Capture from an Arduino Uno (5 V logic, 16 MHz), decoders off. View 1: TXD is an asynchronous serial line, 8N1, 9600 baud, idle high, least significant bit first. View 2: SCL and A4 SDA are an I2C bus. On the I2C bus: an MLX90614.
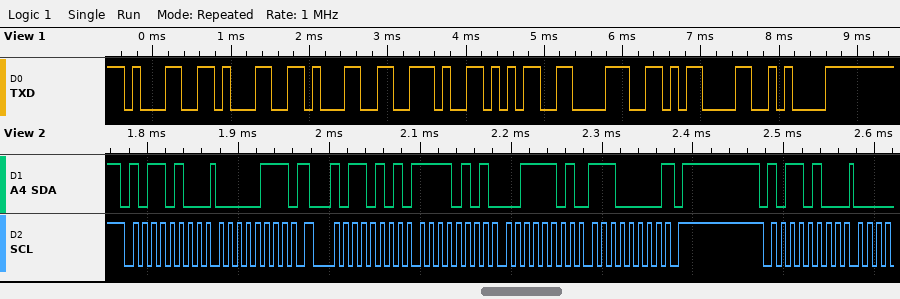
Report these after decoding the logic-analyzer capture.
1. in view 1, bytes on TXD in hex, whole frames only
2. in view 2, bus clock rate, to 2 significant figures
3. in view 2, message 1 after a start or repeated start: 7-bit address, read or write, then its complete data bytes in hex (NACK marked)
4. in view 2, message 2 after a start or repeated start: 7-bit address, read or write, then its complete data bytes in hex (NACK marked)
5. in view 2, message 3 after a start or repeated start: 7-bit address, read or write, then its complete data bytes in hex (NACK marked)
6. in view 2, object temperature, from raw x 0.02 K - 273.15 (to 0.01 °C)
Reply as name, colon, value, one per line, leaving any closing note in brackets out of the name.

in view 1, bytes on TXD in hex, whole frames only: 31 31 31 2E 35 38 0D 0A
in view 2, bus clock rate, to 2 significant figures: 100 kHz
in view 2, message 1 after a start or repeated start: 7-bit address, read or write, then its complete data bytes in hex: 0x5A write: 07
in view 2, message 2 after a start or repeated start: 7-bit address, read or write, then its complete data bytes in hex: 0x5A read: F5 3D E0 NACK
in view 2, message 3 after a start or repeated start: 7-bit address, read or write, then its complete data bytes in hex: 0x5A write
in view 2, object temperature, from raw x 0.02 K - 273.15: 44.07 °C
